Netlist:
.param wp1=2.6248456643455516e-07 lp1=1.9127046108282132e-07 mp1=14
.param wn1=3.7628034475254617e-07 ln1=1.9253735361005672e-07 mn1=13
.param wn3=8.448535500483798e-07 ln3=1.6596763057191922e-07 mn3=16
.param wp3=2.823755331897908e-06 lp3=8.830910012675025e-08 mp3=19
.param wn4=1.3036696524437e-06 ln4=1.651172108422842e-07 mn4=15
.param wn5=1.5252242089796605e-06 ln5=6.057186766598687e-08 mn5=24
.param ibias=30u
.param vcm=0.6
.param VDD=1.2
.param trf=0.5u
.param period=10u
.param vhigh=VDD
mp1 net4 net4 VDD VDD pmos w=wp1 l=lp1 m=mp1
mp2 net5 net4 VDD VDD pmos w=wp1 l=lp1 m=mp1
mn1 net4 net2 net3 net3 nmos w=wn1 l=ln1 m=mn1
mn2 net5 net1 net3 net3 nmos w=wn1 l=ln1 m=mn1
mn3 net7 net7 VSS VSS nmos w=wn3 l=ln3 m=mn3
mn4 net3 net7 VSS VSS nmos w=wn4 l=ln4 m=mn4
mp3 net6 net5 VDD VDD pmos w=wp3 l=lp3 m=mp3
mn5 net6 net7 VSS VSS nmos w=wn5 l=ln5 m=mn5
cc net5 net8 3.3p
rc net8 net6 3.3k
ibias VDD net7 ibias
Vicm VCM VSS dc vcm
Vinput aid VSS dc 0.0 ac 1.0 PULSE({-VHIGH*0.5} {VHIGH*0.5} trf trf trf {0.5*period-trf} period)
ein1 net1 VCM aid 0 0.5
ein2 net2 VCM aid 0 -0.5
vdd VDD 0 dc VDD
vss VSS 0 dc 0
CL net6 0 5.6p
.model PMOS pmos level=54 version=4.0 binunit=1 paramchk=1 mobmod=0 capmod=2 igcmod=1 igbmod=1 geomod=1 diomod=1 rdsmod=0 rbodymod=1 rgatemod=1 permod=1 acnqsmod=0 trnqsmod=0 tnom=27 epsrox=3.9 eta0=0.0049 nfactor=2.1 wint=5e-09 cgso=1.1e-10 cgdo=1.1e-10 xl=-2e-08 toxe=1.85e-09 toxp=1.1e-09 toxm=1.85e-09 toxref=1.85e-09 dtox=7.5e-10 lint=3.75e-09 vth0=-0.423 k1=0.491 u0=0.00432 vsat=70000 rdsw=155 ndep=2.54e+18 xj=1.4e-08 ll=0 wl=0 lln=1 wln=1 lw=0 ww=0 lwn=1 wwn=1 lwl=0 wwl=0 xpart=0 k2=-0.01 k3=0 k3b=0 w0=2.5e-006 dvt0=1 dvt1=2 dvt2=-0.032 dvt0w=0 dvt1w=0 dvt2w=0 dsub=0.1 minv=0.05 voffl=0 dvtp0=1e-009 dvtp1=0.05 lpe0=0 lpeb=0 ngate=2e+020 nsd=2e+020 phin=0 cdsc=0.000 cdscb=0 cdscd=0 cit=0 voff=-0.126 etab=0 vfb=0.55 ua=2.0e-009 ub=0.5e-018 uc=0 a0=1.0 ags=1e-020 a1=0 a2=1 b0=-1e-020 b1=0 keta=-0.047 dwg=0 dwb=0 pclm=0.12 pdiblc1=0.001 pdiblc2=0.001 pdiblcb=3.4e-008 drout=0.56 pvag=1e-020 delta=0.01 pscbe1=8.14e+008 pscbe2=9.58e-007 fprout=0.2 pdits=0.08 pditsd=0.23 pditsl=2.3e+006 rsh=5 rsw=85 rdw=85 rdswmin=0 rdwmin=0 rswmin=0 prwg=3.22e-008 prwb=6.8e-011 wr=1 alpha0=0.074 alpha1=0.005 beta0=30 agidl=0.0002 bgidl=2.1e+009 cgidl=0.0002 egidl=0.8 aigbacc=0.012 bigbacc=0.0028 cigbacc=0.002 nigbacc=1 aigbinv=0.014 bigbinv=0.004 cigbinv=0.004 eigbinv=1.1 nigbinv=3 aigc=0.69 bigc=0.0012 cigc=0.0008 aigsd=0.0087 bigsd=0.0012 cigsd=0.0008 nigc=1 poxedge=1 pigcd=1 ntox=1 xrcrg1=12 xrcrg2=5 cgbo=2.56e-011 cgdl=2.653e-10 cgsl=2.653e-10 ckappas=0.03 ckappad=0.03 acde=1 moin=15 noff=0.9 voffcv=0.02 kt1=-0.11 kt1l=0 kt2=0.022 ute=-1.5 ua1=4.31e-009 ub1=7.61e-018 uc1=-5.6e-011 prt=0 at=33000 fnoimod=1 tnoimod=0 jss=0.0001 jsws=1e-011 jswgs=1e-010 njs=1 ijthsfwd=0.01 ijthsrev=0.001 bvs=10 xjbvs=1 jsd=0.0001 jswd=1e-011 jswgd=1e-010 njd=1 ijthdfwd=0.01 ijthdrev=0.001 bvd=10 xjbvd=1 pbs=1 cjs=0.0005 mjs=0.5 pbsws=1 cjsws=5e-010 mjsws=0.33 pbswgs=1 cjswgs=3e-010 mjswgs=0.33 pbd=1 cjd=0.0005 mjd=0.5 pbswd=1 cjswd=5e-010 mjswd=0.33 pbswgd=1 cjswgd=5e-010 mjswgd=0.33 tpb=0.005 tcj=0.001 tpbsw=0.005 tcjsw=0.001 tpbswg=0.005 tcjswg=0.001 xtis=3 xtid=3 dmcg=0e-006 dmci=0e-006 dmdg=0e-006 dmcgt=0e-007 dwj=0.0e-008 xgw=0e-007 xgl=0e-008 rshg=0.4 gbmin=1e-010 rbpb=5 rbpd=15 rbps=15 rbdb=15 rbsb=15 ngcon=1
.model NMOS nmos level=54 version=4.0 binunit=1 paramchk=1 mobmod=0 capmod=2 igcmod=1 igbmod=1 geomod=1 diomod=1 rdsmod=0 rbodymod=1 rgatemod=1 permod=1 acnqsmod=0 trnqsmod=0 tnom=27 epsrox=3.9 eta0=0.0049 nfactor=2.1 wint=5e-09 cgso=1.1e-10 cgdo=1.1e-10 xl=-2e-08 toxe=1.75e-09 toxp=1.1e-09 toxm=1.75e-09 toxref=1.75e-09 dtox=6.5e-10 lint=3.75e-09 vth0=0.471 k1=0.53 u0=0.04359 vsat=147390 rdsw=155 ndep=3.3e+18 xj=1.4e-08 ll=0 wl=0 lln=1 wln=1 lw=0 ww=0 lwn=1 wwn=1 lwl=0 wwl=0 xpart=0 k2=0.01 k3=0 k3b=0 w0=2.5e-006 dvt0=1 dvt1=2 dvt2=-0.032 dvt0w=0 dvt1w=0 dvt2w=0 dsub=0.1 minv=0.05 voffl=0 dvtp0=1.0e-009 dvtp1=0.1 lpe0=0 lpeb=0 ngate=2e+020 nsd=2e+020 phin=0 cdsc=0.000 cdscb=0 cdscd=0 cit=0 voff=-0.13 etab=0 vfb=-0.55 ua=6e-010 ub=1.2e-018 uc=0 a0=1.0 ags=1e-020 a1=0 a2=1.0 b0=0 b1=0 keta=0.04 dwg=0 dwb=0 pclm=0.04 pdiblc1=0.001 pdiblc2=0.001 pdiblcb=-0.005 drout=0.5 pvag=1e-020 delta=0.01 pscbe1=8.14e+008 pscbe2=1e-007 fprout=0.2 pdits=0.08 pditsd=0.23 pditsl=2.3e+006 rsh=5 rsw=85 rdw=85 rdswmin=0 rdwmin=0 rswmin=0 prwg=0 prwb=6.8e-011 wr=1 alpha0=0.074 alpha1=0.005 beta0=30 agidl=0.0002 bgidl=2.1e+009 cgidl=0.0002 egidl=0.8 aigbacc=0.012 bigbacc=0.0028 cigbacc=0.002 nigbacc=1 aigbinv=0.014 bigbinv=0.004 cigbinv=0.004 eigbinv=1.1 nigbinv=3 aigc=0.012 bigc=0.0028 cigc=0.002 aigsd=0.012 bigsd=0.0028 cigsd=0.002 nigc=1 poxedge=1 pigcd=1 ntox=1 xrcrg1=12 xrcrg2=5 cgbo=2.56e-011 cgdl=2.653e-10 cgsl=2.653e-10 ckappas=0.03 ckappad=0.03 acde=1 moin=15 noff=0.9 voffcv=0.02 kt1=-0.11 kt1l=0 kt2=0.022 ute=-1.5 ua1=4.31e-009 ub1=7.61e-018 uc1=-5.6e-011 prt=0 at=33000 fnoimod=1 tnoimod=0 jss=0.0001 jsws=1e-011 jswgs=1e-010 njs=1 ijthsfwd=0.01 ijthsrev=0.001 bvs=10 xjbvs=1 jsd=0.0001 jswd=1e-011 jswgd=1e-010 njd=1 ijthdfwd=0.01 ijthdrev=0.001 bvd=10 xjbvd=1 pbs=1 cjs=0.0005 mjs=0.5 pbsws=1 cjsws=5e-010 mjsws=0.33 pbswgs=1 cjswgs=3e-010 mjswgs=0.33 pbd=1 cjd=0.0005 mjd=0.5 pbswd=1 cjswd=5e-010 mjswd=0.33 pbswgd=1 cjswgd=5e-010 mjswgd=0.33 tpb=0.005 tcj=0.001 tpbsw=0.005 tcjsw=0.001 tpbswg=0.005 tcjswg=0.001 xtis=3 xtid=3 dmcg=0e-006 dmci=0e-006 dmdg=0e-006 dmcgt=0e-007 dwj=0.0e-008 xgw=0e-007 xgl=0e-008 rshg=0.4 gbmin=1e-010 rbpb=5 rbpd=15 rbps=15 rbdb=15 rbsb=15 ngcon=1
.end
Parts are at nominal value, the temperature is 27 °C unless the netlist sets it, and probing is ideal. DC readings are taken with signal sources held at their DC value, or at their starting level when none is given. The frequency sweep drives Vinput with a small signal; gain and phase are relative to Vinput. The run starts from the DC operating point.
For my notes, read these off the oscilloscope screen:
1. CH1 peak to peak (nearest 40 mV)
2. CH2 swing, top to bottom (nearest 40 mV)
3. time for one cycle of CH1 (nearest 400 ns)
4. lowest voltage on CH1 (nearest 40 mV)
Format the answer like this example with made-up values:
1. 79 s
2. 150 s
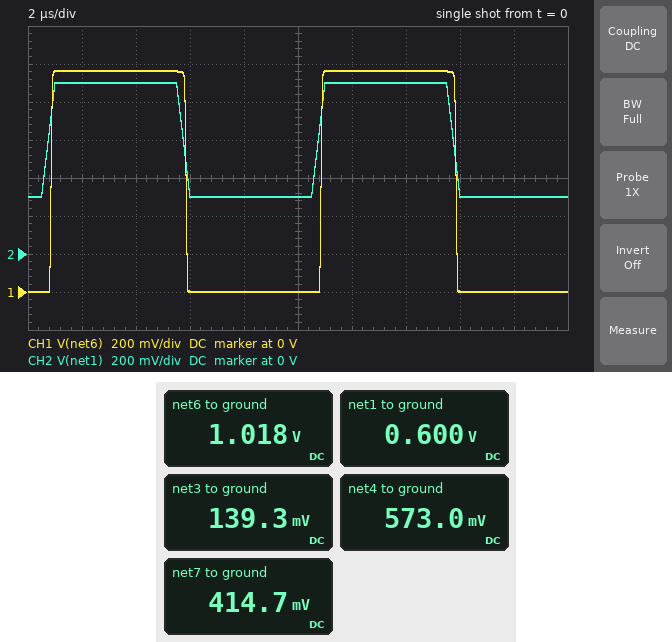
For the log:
1. 1.16 V
2. 600 mV
3. 10.0 µs
4. 0 V
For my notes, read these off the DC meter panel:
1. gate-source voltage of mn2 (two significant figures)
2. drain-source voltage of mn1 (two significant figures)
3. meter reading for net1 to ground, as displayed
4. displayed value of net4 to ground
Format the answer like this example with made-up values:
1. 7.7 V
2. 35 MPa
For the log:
1. 460 mV
2. 430 mV
3. 0.600 V
4. 573.0 mV
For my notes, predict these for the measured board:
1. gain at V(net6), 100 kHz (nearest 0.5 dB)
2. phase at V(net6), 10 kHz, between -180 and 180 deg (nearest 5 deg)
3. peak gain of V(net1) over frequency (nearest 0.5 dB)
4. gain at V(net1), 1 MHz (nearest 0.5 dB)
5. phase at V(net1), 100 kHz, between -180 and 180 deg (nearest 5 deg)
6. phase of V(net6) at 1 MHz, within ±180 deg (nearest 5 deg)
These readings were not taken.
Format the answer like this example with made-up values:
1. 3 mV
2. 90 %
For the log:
1. 41.5 dB
2. -15 deg
3. -6.0 dB
4. -6.0 dB
5. 0 deg
6. -85 deg
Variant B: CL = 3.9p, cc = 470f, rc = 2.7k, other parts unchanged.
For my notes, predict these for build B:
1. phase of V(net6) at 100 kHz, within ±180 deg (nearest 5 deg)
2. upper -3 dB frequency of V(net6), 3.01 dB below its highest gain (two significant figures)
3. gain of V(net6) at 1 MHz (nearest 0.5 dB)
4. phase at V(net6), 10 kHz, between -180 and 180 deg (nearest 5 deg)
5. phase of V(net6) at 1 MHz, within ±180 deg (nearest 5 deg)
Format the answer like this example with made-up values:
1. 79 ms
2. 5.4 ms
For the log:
1. -20 deg
2. 280 kHz
3. 38.0 dB
4. 0 deg
5. -75 deg
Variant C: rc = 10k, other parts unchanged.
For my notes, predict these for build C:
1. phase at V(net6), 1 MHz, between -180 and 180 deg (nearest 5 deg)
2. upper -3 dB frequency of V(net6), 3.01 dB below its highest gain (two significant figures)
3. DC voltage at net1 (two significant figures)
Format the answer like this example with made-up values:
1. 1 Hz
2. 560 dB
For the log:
1. -75 deg
2. 43 kHz
3. 600 mV
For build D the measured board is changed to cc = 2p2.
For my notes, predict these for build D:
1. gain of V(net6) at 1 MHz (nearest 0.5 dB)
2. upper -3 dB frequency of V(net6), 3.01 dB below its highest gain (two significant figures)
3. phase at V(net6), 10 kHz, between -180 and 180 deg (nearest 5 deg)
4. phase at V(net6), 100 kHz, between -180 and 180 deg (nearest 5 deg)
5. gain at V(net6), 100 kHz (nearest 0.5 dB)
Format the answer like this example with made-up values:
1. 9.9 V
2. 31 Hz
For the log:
1. 25.5 dB
2. 65 kHz
3. -10 deg
4. -55 deg
5. 44.0 dB
